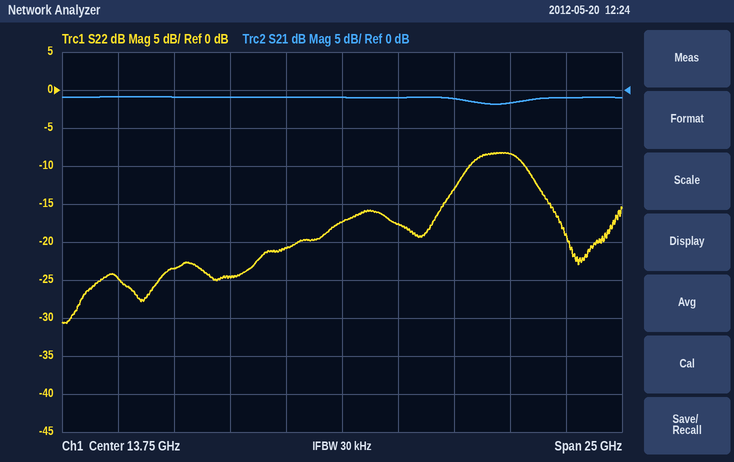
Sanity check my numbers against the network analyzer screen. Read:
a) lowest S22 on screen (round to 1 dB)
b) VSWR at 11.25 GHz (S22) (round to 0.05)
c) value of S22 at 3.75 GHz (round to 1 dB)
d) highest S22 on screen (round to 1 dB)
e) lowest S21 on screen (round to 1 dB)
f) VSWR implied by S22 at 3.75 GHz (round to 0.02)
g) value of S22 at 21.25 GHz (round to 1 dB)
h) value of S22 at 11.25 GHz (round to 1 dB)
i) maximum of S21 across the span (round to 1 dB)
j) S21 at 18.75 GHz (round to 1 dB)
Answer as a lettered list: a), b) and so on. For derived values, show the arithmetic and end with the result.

a) -31 dB
b) |Γ| = 10^(-21/20) = 0.0891; VSWR = (1 + 0.0891)/(1 − 0.0891) ≈ 1.20
c) -25 dB
d) -8 dB
e) -2 dB
f) |Γ| = 10^(-25/20) = 0.0562; VSWR = (1 + 0.0562)/(1 − 0.0562) ≈ 1.12
g) -8 dB
h) -21 dB
i) -1 dB
j) -1 dB
